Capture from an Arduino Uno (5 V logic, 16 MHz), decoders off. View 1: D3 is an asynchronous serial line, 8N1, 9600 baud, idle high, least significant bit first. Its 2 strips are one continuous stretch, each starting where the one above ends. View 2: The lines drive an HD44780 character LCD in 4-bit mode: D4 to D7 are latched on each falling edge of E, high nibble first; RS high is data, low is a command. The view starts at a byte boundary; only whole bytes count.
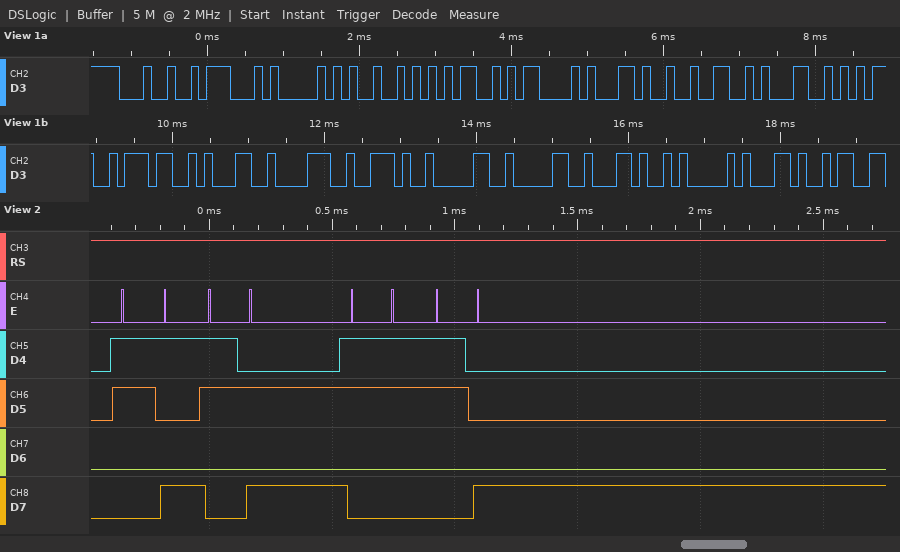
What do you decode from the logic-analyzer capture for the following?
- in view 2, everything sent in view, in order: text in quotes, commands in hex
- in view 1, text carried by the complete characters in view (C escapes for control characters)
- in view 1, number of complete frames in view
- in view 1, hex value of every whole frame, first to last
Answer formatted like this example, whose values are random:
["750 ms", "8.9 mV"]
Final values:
["\"9:38\"", "\"$GPRMC,215718.00,A,\"", "19", "24 47 50 52 4D 43 2C 32 31 35 37 31 38 2E 30 30 2C 41 2C"]
